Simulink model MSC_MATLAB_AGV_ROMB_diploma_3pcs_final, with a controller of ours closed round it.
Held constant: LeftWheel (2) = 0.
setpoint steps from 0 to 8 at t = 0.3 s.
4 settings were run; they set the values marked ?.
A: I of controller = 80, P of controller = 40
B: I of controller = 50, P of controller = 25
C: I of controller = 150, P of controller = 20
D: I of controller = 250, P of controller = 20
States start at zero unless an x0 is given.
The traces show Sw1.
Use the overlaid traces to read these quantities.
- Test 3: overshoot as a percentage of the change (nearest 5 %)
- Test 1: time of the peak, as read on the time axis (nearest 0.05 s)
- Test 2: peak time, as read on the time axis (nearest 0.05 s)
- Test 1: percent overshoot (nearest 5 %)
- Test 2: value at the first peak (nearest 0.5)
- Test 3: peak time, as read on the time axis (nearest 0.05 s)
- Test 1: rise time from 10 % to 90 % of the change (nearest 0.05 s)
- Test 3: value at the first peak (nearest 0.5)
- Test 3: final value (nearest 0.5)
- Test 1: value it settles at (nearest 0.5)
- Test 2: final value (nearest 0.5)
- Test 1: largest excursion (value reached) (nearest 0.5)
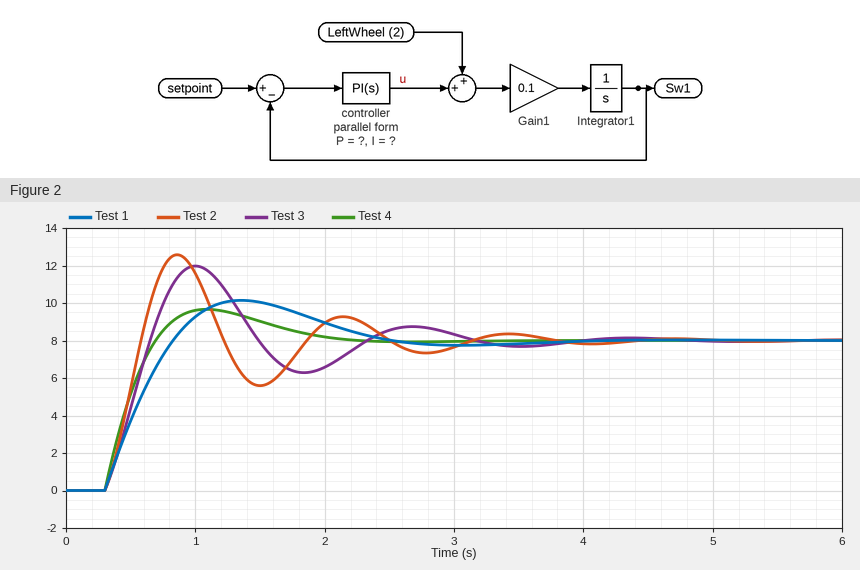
50 %
1.35 s
0.85 s
25 %
12.5
1.00 s
0.40 s
12.0
8.0
8.0
8.0
10.0
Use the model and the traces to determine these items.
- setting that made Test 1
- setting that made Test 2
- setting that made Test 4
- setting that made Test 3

B
D
A
C
